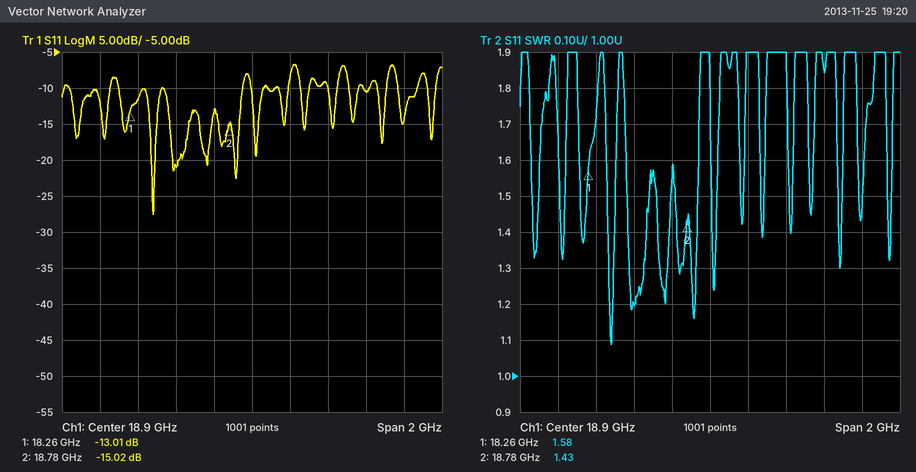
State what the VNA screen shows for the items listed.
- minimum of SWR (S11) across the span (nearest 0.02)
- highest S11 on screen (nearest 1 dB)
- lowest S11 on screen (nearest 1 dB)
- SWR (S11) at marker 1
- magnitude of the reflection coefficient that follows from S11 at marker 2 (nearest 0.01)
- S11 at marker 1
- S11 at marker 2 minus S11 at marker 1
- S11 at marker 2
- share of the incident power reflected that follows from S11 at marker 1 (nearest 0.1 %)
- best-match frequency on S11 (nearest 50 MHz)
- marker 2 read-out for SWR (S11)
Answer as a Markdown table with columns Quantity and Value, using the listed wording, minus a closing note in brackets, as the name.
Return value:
| Quantity | Value |
|---|---|
| minimum of SWR (S11) across the span | 1.08 |
| highest S11 on screen | -7 dB |
| lowest S11 on screen | -28 dB |
| SWR (S11) at marker 1 | 1.58 |
| magnitude of the reflection coefficient that follows from S11 at marker 2 | 0.18 |
| S11 at marker 1 | -13.01 dB |
| S11 at marker 2 minus S11 at marker 1 | -2.01 dB |
| S11 at marker 2 | -15.02 dB |
| share of the incident power reflected that follows from S11 at marker 1 | 5.0 % |
| best-match frequency on S11 | 18.40 GHz |
| marker 2 read-out for SWR | 1.43 |
